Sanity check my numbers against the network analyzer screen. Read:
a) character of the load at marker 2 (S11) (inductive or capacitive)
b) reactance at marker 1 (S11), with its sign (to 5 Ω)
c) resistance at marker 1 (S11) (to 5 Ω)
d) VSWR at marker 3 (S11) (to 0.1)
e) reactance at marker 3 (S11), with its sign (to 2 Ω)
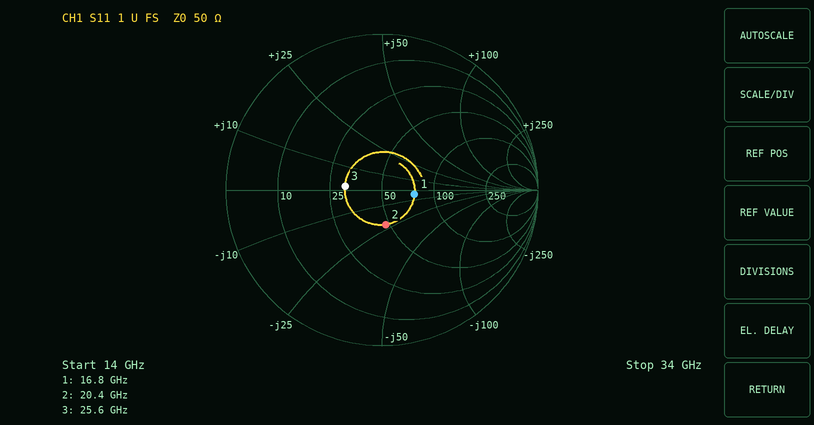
capacitive
-5 Ω
75 Ω
1.6
+2 Ω
